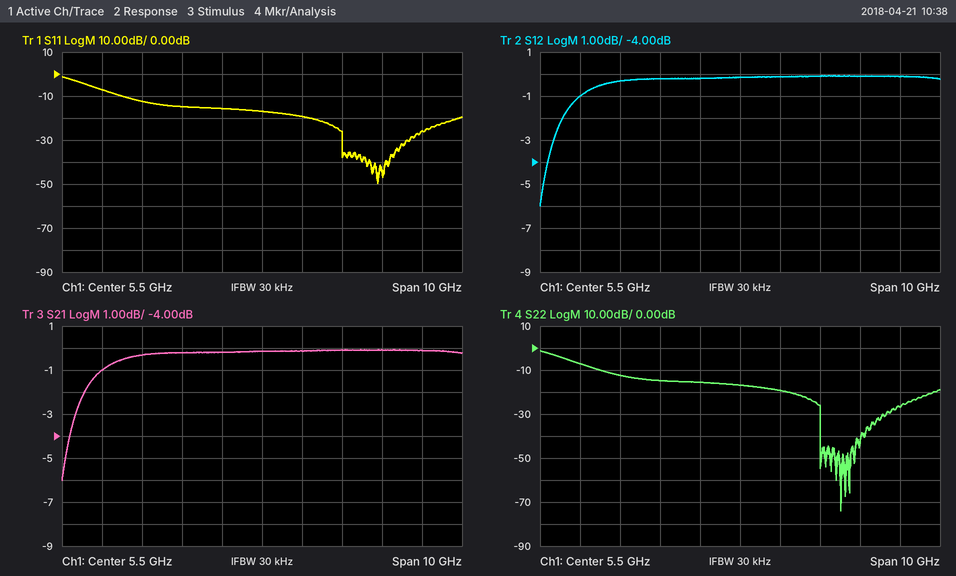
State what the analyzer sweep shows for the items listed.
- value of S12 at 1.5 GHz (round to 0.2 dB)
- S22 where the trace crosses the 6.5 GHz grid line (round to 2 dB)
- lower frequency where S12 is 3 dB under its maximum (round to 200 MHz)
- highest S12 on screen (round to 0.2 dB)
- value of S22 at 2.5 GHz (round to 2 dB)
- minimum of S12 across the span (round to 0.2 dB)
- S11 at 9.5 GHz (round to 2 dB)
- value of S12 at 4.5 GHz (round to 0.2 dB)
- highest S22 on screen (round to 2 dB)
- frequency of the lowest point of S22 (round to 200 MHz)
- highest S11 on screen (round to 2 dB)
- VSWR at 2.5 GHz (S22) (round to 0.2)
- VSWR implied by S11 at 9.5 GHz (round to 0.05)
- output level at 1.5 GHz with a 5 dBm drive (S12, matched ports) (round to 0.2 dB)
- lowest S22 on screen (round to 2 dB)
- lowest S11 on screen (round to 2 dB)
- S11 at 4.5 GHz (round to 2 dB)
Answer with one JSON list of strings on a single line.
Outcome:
["-1.0 dB", "-20 dB", "800 MHz", "0.0 dB", "-12 dB", "-6.0 dB", "-26 dB", "-0.2 dB", "-2 dB", "8.0 GHz", "-2 dB", "1.6", "1.10", "4.0 dBm", "-74 dB", "-50 dB", "-16 dB"]
